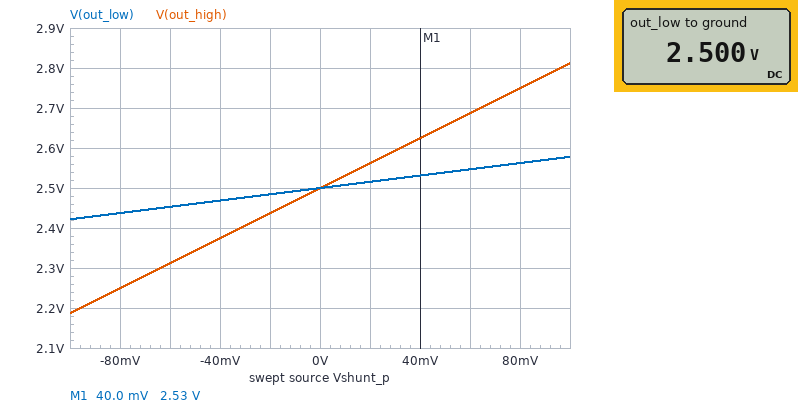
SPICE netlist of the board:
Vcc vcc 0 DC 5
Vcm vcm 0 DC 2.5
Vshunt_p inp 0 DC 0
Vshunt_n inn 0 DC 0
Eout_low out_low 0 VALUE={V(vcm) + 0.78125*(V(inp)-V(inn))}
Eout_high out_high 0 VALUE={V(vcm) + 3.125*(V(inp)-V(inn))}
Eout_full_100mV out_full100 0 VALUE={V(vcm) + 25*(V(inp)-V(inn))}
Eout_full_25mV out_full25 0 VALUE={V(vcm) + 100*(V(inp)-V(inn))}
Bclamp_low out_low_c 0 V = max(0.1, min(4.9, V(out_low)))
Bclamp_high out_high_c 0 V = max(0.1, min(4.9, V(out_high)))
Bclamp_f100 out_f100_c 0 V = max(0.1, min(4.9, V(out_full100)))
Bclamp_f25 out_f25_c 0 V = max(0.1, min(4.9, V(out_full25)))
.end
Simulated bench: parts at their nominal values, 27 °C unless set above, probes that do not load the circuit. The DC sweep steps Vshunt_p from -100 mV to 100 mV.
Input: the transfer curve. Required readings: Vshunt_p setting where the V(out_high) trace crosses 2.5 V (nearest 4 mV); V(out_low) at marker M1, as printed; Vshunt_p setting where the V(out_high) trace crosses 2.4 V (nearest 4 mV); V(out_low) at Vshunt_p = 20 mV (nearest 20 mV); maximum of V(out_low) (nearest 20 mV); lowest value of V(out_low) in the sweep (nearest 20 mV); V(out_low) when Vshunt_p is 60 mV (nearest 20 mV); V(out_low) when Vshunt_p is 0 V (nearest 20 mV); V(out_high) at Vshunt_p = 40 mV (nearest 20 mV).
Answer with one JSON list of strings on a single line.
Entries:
["0 V", "2.53 V", "-32 mV", "2.52 V", "2.58 V", "2.42 V", "2.54 V", "2.50 V", "2.62 V"]
